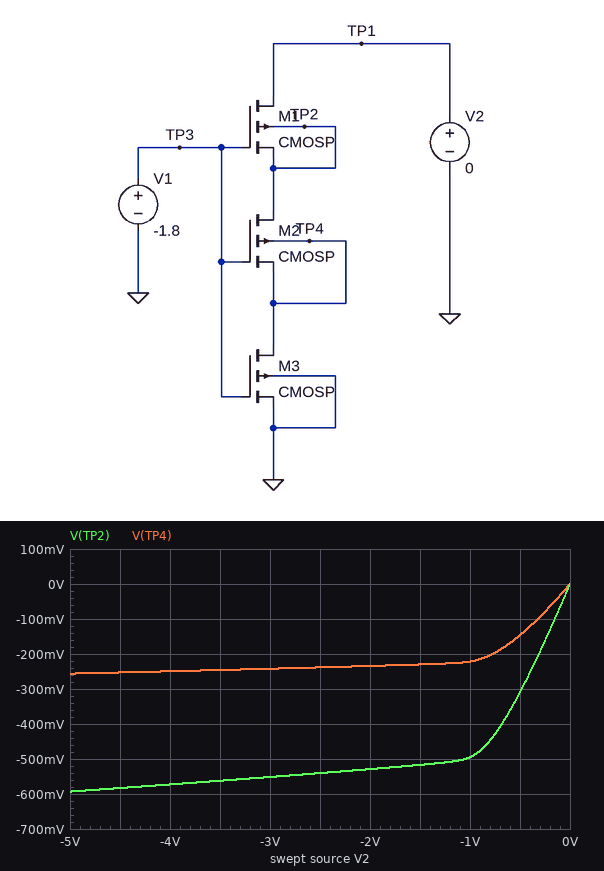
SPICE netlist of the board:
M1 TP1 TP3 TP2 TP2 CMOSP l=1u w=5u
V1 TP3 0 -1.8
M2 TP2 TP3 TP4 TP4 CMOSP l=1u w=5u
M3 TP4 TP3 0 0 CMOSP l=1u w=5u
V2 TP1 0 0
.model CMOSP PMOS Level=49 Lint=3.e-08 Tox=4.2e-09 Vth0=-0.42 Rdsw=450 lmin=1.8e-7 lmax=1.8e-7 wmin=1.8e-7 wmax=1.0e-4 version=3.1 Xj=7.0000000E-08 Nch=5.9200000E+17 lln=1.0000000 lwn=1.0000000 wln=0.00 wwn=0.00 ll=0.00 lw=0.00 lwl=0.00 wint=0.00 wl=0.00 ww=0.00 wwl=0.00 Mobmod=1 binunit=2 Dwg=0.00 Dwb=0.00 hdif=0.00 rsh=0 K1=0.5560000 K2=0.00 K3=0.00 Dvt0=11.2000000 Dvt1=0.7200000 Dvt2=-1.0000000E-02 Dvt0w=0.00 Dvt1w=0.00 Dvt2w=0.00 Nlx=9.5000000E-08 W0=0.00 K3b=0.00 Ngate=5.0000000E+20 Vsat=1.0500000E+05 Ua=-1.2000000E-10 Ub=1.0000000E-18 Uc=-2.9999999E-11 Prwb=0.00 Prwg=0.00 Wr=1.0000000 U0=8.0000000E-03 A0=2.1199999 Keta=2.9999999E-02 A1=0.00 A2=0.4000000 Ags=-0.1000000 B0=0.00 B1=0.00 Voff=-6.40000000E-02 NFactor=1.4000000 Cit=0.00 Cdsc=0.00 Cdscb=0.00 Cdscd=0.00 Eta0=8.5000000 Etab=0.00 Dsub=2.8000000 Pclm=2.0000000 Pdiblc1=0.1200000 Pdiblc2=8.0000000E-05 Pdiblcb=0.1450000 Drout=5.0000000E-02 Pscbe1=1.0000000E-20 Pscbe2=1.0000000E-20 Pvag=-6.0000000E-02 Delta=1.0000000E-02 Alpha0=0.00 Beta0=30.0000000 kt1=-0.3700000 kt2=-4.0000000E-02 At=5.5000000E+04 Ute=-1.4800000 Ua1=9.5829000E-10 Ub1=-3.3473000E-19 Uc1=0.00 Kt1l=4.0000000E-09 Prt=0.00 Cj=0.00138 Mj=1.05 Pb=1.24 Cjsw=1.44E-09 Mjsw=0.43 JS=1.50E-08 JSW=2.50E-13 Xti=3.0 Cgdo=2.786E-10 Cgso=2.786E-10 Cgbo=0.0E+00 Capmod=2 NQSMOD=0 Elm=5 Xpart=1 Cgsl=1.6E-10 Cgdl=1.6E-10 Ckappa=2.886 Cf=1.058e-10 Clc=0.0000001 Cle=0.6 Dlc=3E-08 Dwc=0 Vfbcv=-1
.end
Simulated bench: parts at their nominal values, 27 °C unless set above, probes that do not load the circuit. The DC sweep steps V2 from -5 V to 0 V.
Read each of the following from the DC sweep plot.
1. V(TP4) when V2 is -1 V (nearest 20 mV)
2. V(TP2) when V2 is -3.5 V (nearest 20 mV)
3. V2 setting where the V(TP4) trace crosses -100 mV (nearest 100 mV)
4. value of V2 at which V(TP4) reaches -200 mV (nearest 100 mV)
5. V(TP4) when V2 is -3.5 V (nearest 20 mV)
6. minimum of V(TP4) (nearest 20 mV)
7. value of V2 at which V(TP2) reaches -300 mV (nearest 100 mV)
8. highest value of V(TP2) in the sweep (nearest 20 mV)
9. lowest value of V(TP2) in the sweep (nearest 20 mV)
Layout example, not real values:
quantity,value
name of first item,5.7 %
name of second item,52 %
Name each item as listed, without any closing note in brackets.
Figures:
quantity,value
V(TP4) when V2 is -1 V,-220 mV
V(TP2) when V2 is -3.5 V,-560 mV
V2 setting where the V(TP4) trace crosses -100 mV,-300 mV
value of V2 at which V(TP4) reaches -200 mV,-800 mV
V(TP4) when V2 is -3.5 V,-240 mV
minimum of V(TP4),-260 mV
value of V2 at which V(TP2) reaches -300 mV,-500 mV
highest value of V(TP2) in the sweep,0 V
lowest value of V(TP2) in the sweep,-600 mV
